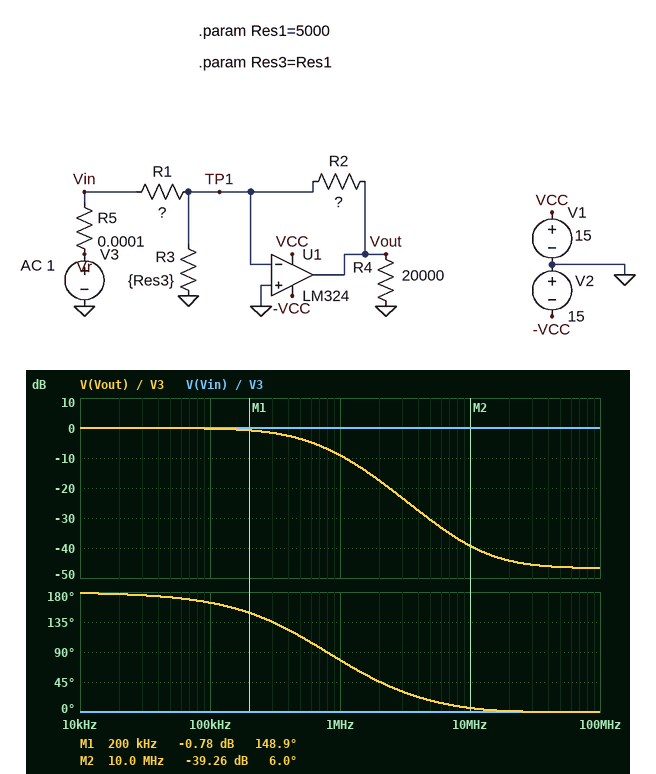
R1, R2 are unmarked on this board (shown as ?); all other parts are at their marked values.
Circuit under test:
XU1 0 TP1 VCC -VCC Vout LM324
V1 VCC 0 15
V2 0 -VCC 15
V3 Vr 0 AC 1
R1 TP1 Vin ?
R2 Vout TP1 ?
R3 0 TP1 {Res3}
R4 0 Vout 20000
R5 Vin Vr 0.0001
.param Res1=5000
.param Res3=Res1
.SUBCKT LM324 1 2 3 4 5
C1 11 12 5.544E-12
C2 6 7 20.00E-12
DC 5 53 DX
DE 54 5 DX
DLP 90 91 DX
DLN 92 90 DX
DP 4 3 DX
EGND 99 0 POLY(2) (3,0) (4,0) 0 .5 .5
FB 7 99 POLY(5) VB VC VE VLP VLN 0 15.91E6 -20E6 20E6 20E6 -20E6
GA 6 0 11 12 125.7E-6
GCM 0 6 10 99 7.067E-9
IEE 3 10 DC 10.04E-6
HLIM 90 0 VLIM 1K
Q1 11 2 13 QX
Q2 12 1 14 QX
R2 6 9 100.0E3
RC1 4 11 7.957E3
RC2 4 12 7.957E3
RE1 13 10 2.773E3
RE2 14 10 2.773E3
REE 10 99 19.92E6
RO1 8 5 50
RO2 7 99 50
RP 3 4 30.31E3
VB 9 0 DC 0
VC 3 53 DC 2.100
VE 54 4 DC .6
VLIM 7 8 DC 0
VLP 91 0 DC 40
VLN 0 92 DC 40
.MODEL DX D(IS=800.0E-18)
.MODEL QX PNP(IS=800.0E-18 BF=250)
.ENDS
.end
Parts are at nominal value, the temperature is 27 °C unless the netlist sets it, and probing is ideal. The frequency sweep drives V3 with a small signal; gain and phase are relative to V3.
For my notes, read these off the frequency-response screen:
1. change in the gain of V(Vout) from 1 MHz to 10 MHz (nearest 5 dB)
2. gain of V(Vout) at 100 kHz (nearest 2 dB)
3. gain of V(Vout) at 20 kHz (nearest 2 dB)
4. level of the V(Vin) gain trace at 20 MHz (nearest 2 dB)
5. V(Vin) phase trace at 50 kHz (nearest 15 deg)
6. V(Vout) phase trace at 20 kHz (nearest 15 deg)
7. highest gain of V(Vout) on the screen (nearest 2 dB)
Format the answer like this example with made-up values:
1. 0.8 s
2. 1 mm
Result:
1. -30 dB
2. 0 dB
3. 0 dB
4. 0 dB
5. 0 deg
6. 180 deg
7. 0 dB
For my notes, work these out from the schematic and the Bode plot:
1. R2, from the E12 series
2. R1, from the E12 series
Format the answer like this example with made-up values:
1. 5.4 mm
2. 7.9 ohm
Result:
1. 3.9 kΩ
2. 3.9 kΩ
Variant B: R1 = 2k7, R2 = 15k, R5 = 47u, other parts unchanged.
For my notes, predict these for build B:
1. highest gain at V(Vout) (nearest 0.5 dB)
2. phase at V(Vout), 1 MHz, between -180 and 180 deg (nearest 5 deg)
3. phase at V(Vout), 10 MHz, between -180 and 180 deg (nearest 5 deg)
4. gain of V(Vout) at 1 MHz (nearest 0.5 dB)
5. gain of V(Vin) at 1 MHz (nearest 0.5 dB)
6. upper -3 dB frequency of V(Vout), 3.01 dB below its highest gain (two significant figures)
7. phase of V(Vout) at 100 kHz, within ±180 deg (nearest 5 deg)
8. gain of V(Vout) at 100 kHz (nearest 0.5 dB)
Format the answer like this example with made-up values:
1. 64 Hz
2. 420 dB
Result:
1. 15.0 dB
2. 65 deg
3. 10 deg
4. -5.5 dB
5. 0 dB
6. 110 kHz
7. 135 deg
8. 12.5 dB
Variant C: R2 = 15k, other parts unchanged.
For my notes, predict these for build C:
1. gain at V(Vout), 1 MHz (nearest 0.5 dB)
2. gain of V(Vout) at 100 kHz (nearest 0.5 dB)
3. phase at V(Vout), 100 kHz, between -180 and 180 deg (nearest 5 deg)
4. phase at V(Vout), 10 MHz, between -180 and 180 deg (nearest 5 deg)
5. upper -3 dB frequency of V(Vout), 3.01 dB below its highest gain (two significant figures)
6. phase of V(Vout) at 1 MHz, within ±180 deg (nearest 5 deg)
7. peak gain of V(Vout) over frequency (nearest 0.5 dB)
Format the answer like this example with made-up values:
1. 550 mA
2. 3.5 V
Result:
1. -7.0 dB
2. 10.0 dB
3. 140 deg
4. 10 deg
5. 140 kHz
6. 65 deg
7. 11.5 dB
